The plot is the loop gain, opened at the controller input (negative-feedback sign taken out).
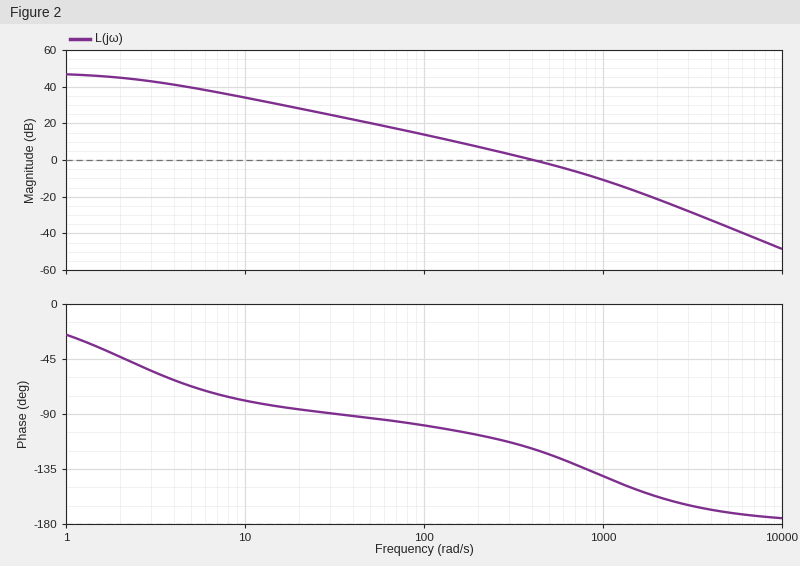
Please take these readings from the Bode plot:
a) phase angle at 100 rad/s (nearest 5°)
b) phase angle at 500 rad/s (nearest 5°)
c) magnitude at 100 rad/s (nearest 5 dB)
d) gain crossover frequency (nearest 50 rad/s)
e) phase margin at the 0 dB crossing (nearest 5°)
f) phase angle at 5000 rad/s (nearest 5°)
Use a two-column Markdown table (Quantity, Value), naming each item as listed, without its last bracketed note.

| Quantity | Value |
|---|---|
| phase angle at 100 rad/s | -100° |
| phase angle at 500 rad/s | -125° |
| magnitude at 100 rad/s | 15 dB |
| gain crossover frequency | 400 rad/s |
| phase margin at the 0 dB crossing | 60° |
| phase angle at 5000 rad/s | -170° |
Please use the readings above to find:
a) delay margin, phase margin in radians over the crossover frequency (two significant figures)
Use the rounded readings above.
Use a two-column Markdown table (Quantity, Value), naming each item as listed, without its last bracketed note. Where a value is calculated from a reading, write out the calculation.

| Quantity | Value |
|---|---|
| delay margin, phase margin in radians over the crossover frequency | 60 × π / 180 / 400 = 0.0026 s |
